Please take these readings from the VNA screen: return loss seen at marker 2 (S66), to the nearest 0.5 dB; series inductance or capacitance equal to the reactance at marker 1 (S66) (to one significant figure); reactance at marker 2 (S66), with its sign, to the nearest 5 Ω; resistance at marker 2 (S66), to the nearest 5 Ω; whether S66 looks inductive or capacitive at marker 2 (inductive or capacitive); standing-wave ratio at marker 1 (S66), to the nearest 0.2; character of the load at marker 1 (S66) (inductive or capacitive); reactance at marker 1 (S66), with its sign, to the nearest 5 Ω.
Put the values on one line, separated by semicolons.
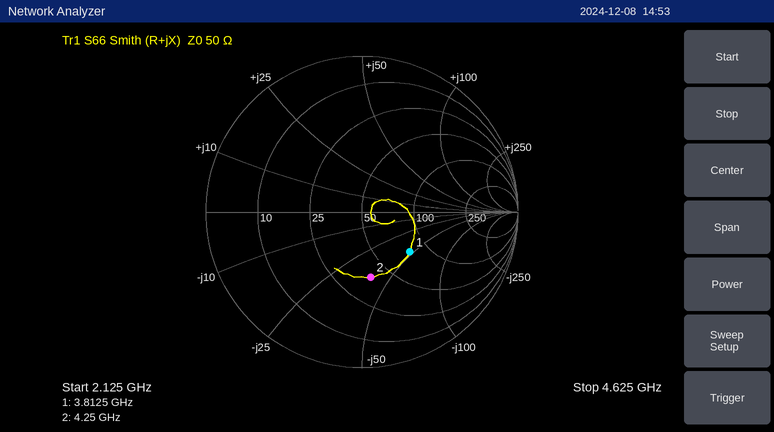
7.5 dB; 900 fF; -40 Ω; 40 Ω; capacitive; 2.4; capacitive; -45 Ω
